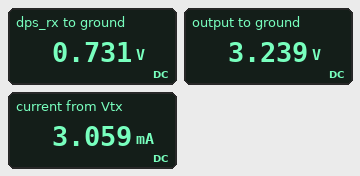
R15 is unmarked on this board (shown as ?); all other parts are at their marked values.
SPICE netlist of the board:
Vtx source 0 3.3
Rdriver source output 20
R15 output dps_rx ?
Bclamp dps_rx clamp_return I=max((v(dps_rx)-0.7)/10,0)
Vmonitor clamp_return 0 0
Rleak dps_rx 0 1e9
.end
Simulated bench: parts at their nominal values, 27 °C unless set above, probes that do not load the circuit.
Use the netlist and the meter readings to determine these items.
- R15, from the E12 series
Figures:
820 Ω
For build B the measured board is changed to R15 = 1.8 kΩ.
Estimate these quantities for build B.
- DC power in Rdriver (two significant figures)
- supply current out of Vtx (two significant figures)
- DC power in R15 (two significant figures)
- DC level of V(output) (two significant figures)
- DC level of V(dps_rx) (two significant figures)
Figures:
40 µW
1.4 mA
3.6 mW
3.3 V
710 mV
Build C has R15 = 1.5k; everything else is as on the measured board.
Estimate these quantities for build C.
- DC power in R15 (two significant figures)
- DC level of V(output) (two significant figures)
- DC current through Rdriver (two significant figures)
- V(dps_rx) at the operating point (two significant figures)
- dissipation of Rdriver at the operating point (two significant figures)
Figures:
4.3 mW
3.3 V
1.7 mA
720 mV
58 µW
